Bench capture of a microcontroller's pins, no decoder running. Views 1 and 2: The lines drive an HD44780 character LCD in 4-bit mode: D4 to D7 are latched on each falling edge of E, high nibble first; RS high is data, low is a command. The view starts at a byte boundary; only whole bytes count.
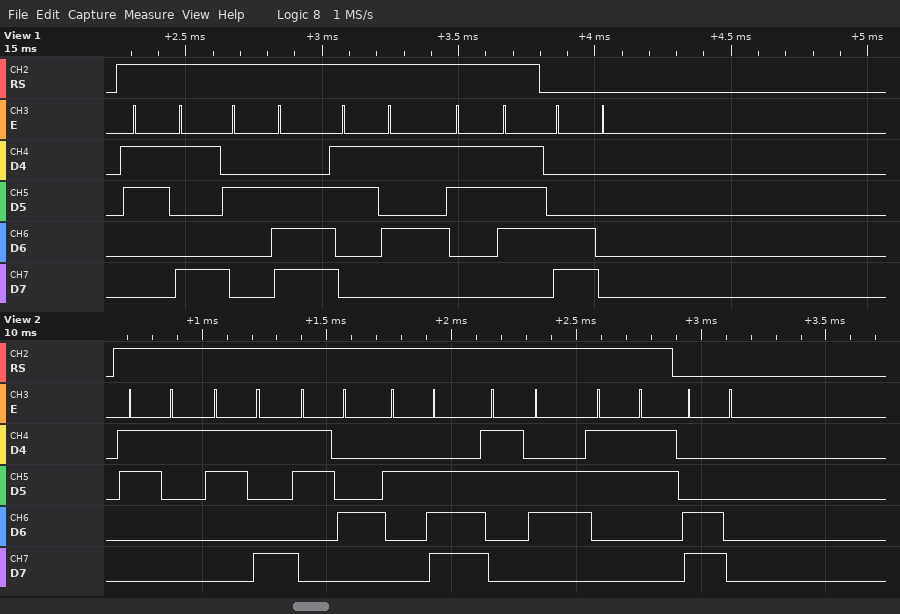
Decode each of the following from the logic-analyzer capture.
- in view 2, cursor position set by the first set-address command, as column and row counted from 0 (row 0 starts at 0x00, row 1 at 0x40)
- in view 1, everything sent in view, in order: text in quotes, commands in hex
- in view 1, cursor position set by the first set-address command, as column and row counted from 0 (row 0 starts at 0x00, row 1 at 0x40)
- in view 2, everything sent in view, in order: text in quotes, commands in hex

column 0, row 1
"9.57" 0xC0
column 0, row 1
"194.63" 0xC0
